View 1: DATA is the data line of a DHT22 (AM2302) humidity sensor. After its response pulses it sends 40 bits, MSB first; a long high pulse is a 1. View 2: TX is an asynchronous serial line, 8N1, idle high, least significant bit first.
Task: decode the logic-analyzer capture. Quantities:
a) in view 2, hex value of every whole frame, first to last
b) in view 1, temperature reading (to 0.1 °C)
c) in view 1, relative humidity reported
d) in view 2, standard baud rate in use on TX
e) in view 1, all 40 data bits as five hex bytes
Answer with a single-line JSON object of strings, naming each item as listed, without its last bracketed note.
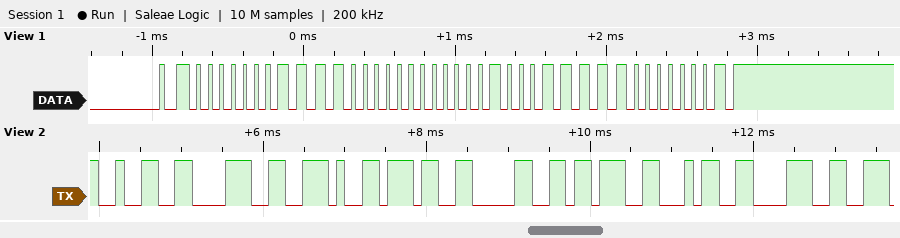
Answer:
{"in view 2, hex value of every whole frame, first to last": "32 38 2E 37 30 3B 34 38", "in view 1, temperature reading": "28.7 °C", "in view 1, relative humidity reported": "48.0 %", "in view 2, standard baud rate in use on TX": "9600 baud", "in view 1, all 40 data bits as five hex bytes": "01 E0 01 1F 01"}
